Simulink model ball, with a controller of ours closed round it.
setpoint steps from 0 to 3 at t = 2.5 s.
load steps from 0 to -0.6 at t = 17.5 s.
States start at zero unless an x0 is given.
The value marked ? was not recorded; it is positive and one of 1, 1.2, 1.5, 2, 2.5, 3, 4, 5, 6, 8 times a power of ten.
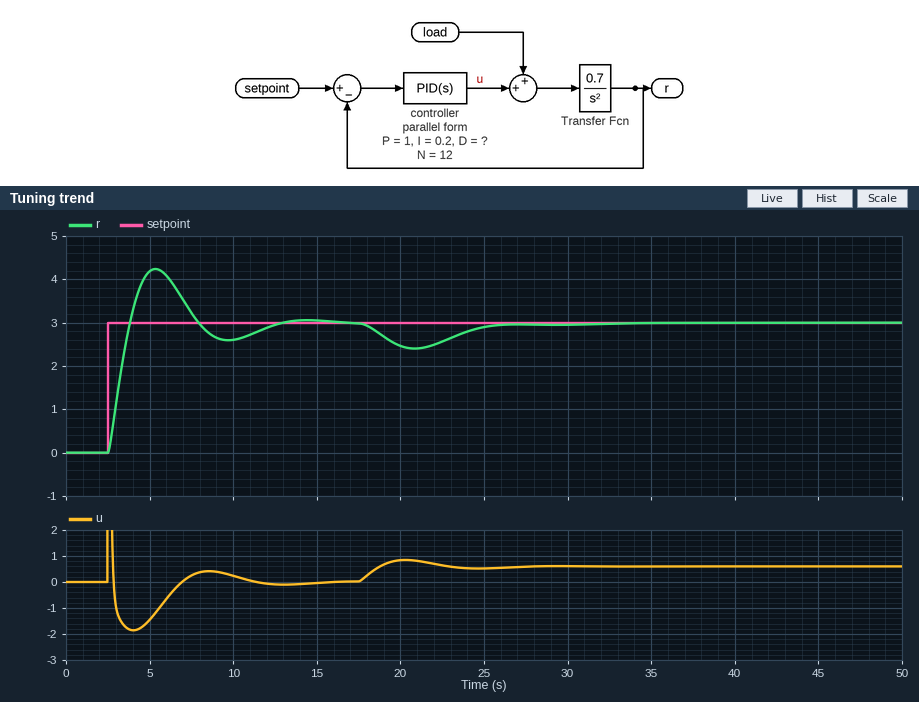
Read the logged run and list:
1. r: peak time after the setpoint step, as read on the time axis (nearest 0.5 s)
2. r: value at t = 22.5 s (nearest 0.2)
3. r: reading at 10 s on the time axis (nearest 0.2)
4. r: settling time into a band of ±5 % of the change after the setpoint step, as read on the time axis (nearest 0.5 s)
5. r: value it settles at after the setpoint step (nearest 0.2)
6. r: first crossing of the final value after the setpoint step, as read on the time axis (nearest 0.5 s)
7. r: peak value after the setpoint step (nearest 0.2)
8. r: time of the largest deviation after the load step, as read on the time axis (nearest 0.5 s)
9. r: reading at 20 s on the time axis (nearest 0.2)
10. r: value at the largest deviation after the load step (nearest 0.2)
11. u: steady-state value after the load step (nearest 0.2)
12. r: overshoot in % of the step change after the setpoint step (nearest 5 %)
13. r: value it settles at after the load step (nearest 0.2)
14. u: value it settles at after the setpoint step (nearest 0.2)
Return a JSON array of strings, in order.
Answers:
["5.5 s", "2.6", "2.6", "12.0 s", "3.0", "4.0 s", "4.2", "21.0 s", "2.4", "2.4", "0.6", "40 %", "3.0", "0.0"]
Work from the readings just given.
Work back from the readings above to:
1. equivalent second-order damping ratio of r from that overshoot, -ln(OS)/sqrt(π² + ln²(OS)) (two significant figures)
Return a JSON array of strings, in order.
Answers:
["0.28"]
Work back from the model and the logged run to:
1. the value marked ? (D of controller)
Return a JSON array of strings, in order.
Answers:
["1.2"]
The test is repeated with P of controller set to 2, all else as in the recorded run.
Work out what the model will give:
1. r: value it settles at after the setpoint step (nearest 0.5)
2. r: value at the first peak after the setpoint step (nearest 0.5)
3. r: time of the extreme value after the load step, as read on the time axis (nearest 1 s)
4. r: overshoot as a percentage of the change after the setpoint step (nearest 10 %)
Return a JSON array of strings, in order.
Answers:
["3.0", "4.5", "20 s", "50 %"]
